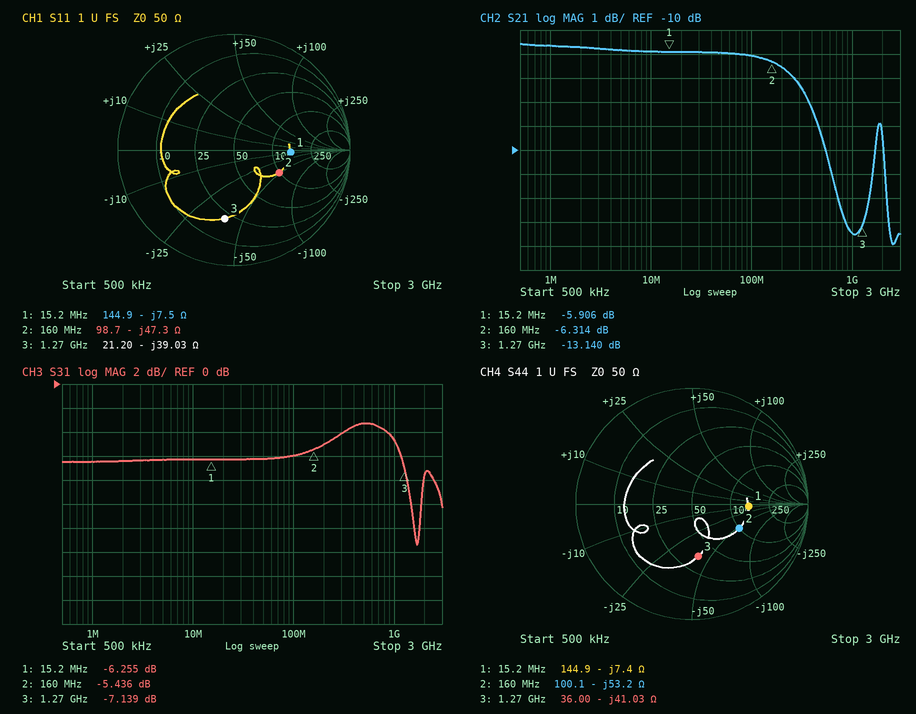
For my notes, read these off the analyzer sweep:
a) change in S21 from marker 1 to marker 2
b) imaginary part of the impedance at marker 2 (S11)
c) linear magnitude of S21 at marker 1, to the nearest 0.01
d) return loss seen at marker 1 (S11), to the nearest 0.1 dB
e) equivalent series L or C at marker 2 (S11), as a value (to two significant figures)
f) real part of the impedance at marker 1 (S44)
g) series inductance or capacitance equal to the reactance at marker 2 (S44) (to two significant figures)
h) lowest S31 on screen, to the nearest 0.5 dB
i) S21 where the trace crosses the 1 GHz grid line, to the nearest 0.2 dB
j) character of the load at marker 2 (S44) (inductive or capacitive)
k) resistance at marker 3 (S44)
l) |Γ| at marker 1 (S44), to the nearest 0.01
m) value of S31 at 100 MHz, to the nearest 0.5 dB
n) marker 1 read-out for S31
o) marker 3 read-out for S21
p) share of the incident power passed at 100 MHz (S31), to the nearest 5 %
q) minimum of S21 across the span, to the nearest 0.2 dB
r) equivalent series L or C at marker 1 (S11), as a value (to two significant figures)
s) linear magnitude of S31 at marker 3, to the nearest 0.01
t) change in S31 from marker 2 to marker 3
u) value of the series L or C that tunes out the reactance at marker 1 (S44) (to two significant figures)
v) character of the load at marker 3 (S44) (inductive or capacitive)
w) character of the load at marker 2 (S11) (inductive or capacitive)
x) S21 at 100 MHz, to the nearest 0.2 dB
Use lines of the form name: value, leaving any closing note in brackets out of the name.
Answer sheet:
change in S21 from marker 1 to marker 2: -0.408 dB
imaginary part of the impedance at marker 2: -47.3 Ω
linear magnitude of S21 at marker 1, to the nearest 0.01: 0.51
return loss seen at marker 1 (S11), to the nearest 0.1 dB: 6.2 dB
equivalent series L or C at marker 2 (S11), as a value: 21 pF
real part of the impedance at marker 1: 144.9 Ω
series inductance or capacitance equal to the reactance at marker 2 (S44): 19 pF
lowest S31 on screen, to the nearest 0.5 dB: -13.5 dB
S21 where the trace crosses the 1 GHz grid line, to the nearest 0.2 dB: -13.4 dB
character of the load at marker 2 (S44): capacitive
resistance at marker 3: 36.00 Ω
|Γ| at marker 1 (S44), to the nearest 0.01: 0.49
value of S31 at 100 MHz, to the nearest 0.5 dB: -6.0 dB
marker 1 read-out for S31: -6.255 dB
marker 3 read-out for S21: -13.140 dB
share of the incident power passed at 100 MHz (S31), to the nearest 5 %: 25 %
minimum of S21 across the span, to the nearest 0.2 dB: -14.0 dB
equivalent series L or C at marker 1 (S11), as a value: 1.4 nF
linear magnitude of S31 at marker 3, to the nearest 0.01: 0.44
change in S31 from marker 2 to marker 3: -1.703 dB
value of the series L or C that tunes out the reactance at marker 1 (S44): 77 nH
character of the load at marker 3 (S44): capacitive
character of the load at marker 2 (S11): capacitive
S21 at 100 MHz, to the nearest 0.2 dB: -6.0 dB
